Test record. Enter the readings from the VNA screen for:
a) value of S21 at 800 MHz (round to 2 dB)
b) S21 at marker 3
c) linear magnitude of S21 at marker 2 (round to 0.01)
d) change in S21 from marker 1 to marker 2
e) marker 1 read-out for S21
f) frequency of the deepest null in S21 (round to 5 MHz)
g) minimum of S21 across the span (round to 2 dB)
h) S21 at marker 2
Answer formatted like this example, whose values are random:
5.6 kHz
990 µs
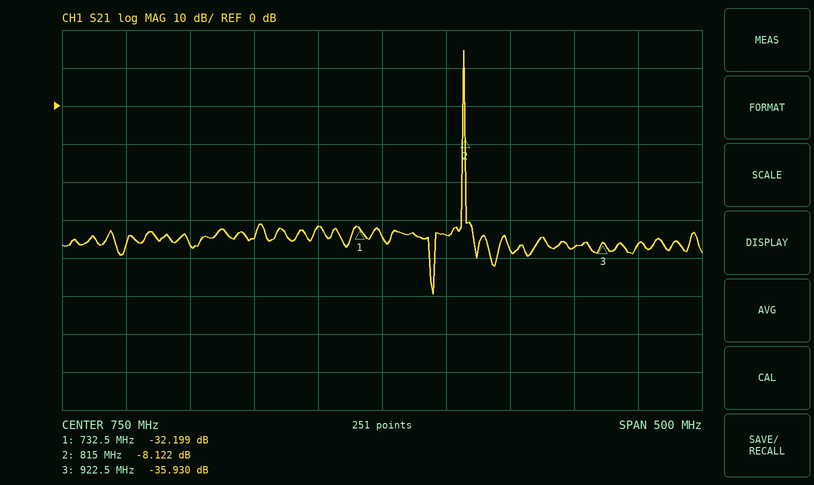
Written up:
-34 dB
-35.930 dB
0.39
24.077 dB
-32.199 dB
790 MHz
-50 dB
-8.122 dB
